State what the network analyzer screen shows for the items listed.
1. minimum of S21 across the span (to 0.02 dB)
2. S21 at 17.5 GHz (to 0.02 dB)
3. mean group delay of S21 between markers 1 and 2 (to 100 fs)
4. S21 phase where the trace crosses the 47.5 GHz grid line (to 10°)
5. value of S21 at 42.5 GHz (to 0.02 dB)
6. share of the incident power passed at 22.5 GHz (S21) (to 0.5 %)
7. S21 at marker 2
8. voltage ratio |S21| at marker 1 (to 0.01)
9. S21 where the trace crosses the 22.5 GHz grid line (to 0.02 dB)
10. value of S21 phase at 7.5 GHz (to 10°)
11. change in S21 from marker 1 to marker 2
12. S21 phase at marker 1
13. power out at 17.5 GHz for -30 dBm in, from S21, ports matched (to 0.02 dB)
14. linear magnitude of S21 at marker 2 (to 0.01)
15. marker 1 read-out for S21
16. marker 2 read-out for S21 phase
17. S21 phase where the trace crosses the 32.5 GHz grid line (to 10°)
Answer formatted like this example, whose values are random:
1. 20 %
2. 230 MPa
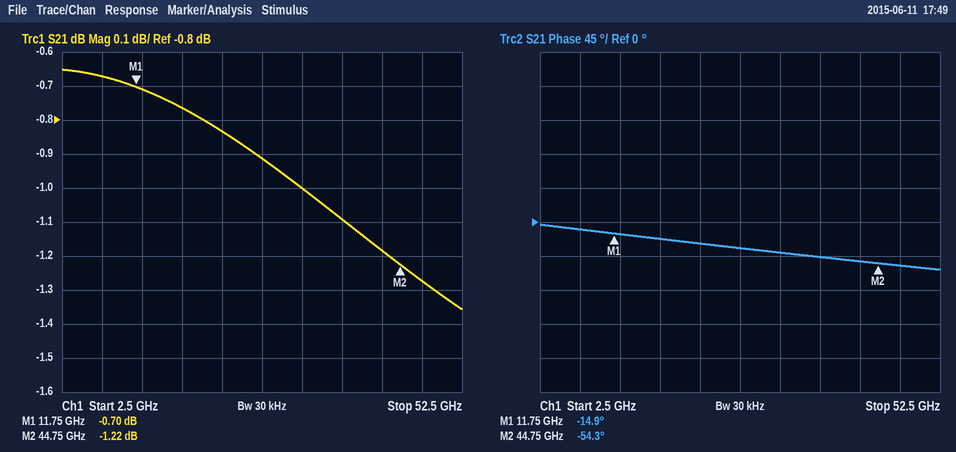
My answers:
1. -1.36 dB
2. -0.76 dB
3. 3.3 ps
4. -60°
5. -1.18 dB
6. 82.5 %
7. -1.22 dB
8. 0.92
9. -0.84 dB
10. -10°
11. -0.52 dB
12. -14.9°
13. -30.76 dBm
14. 0.87
15. -0.70 dB
16. -54.3°
17. -40°
